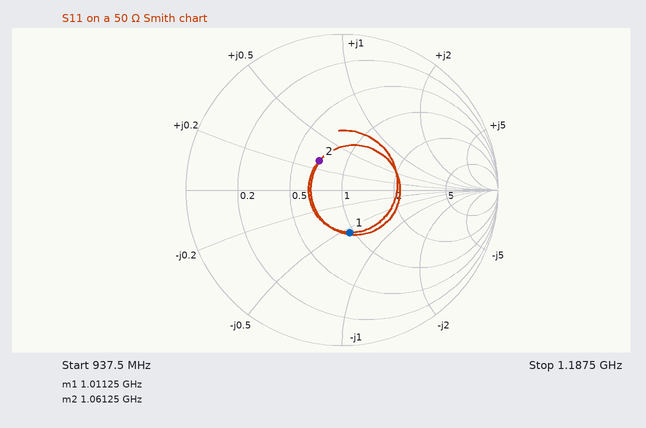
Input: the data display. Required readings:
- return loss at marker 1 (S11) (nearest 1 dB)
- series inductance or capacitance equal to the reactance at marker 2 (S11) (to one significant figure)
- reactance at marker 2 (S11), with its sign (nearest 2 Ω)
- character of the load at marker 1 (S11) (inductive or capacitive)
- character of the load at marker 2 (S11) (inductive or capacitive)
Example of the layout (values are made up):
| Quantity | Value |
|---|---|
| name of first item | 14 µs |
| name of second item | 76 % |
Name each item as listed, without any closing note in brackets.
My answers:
| Quantity | Value |
|---|---|
| return loss at marker 1 (S11) | 11 dB |
| series inductance or capacitance equal to the reactance at marker 2 (S11) | 2 nH |
| reactance at marker 2 (S11), with its sign | +14 Ω |
| character of the load at marker 1 (S11) | capacitive |
| character of the load at marker 2 (S11) | inductive |
